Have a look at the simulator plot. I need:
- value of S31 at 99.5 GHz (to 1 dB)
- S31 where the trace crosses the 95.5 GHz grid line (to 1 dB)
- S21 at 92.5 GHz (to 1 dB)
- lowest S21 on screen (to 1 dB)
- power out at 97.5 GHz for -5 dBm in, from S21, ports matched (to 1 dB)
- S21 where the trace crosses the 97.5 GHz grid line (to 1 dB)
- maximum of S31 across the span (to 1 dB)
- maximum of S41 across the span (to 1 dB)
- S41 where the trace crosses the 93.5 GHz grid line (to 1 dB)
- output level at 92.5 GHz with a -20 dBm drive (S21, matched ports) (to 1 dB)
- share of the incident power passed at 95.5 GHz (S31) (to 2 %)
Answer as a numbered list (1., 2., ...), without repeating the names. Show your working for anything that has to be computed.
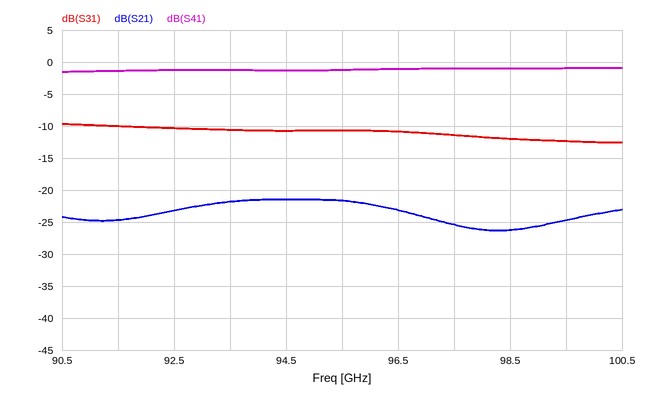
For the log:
1. -12 dB
2. -11 dB
3. -23 dB
4. -26 dB
5. -5 dBm + (-25 dB) = -30 dBm
6. -25 dB
7. -10 dB
8. -1 dB
9. -1 dB
10. -20 dBm + (-23 dB) = -43 dBm
11. 10^(-11/10) ≈ 8 %
